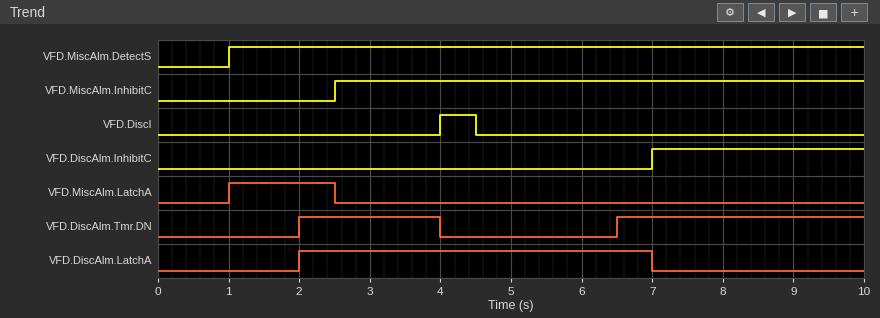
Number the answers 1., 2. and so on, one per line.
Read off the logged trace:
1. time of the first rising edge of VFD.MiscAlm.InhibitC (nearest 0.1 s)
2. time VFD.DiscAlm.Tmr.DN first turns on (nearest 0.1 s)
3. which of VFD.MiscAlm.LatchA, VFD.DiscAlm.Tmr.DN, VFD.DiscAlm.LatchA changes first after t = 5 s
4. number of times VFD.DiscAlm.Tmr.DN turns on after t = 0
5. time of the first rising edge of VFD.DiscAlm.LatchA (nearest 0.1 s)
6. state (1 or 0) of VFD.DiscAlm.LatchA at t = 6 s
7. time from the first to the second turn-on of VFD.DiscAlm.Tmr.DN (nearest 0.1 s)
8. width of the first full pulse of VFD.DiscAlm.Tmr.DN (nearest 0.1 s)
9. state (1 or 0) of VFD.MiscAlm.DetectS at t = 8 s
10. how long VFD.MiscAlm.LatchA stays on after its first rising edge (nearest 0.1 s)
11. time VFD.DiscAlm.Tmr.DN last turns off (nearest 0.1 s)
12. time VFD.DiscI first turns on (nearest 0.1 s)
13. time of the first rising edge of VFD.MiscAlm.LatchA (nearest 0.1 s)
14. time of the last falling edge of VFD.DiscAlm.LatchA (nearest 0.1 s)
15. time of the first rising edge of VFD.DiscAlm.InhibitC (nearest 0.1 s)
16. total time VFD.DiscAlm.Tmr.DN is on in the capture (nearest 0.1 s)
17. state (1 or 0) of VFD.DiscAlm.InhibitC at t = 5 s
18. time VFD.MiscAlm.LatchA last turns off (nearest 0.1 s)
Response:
1. 2.5 s
2. 2.0 s
3. VFD.DiscAlm.Tmr.DN
4. 2
5. 2.0 s
6. 1
7. 4.5 s
8. 2.0 s
9. 1
10. 1.5 s
11. 4.0 s
12. 4.0 s
13. 1.0 s
14. 7.0 s
15. 7.0 s
16. 5.5 s
17. 0
18. 2.5 s
